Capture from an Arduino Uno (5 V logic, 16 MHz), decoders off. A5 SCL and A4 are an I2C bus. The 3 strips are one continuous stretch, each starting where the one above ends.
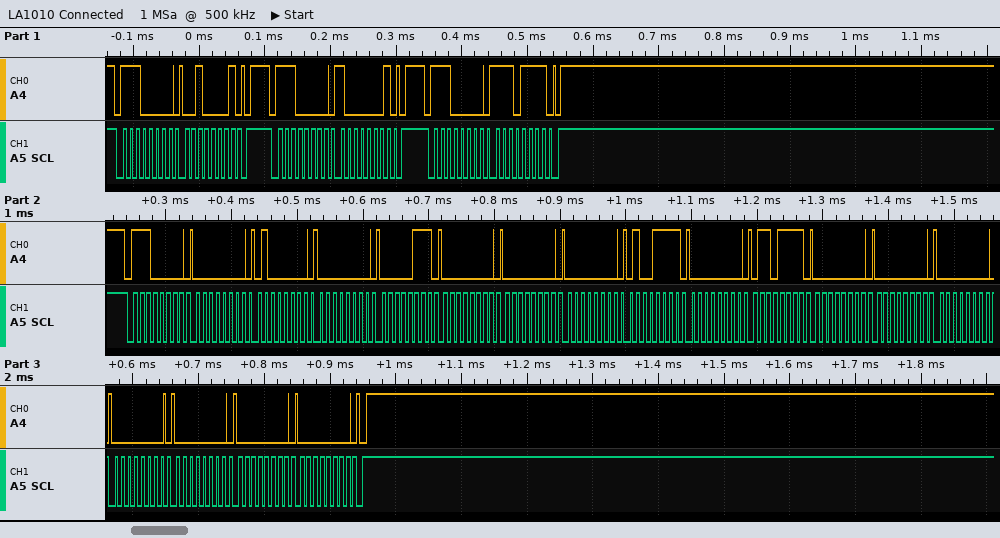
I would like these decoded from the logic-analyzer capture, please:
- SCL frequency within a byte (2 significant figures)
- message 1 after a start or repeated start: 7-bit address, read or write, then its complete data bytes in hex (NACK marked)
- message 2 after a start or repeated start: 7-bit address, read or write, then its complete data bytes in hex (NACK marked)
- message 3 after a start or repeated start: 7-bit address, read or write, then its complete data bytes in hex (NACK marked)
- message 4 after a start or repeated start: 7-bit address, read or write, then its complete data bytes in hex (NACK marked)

100 kHz
0x70 write: 21
0x70 write: 81
0x70 write: EF
0x70 write: 00 40 00 07 00 00 00 4F 00 6F 00 00 00 00 00 00 00
